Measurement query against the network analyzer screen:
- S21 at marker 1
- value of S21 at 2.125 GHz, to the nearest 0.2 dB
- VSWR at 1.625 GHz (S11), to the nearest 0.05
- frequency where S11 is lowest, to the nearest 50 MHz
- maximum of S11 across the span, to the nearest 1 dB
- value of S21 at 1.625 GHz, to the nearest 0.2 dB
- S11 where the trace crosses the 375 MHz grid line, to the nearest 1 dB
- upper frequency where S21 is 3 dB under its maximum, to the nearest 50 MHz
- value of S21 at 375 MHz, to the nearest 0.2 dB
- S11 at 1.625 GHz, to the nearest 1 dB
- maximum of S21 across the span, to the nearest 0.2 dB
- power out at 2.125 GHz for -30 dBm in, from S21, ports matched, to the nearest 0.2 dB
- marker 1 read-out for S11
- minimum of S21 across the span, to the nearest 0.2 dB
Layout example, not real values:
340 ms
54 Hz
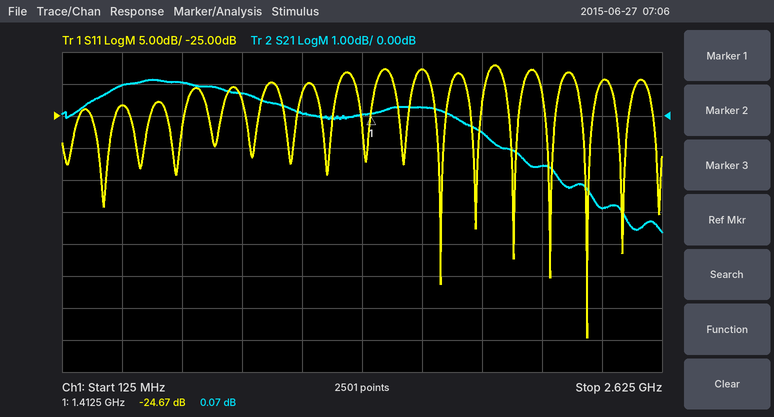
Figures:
0.07 dB
-1.6 dB
1.30
2.30 GHz
-17 dB
0.2 dB
-23 dB
2.20 GHz
1.0 dB
-18 dB
1.2 dB
-31.6 dBm
-24.67 dB
-3.6 dB
